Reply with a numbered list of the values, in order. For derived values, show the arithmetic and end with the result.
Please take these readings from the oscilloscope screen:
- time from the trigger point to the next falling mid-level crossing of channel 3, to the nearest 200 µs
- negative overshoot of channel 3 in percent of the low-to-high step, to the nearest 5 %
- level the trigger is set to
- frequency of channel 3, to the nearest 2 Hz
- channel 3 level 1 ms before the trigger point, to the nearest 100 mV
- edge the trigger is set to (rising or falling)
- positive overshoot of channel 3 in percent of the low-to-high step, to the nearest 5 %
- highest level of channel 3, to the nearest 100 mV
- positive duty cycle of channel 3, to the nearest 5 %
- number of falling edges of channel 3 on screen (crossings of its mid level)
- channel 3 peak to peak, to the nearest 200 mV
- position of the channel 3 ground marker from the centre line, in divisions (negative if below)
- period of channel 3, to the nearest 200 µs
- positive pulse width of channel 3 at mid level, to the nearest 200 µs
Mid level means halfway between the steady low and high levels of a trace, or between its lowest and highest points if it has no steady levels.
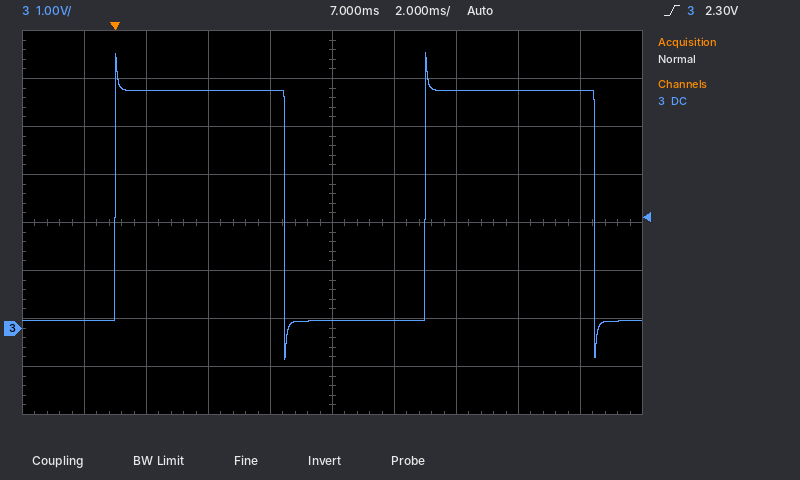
1. 5.4 ms
2. 15 %
3. 2.30 V
4. 1 / 10.0 ms ≈ 100 Hz
5. 200 mV
6. rising
7. 15 %
8. 5.7 V
9. 5.4 ms / 10.0 ms ≈ 54.0 %, so 55 % to the nearest 5 %
10. 2
11. 6.4 V
12. -2.2 div
13. 10.0 ms
14. 5.4 ms
